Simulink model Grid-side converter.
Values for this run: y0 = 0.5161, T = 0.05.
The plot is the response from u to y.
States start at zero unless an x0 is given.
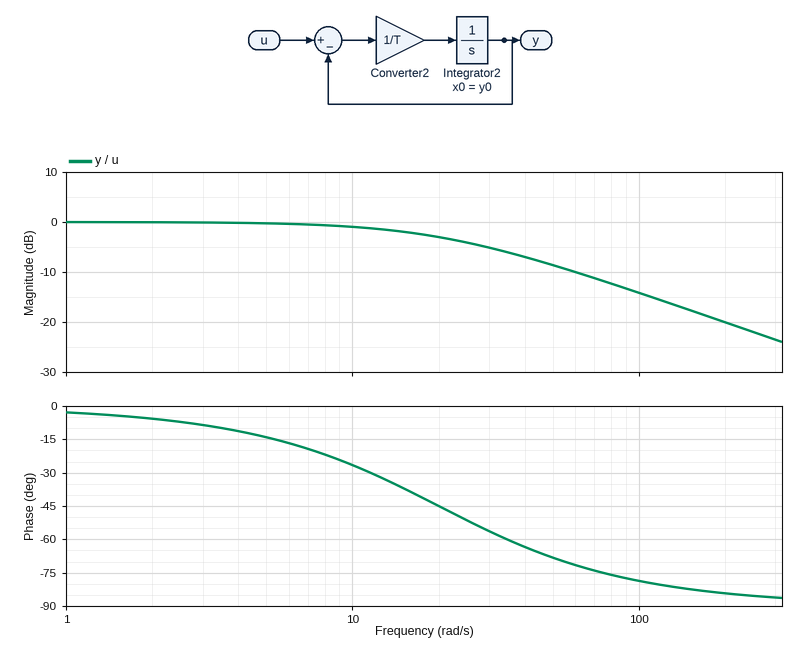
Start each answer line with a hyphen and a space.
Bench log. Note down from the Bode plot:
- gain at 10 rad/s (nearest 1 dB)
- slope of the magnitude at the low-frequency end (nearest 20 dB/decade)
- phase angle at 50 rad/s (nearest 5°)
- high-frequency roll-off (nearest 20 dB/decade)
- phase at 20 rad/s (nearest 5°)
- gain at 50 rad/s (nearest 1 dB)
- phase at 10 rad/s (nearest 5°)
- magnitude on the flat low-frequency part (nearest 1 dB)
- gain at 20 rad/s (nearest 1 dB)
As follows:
- -1 dB
- 0 dB/decade
- -70°
- -20 dB/decade
- -45°
- -9 dB
- -25°
- 0 dB
- -3 dB
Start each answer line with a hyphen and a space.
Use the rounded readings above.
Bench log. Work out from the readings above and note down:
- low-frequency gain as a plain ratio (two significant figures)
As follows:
- 1.0
